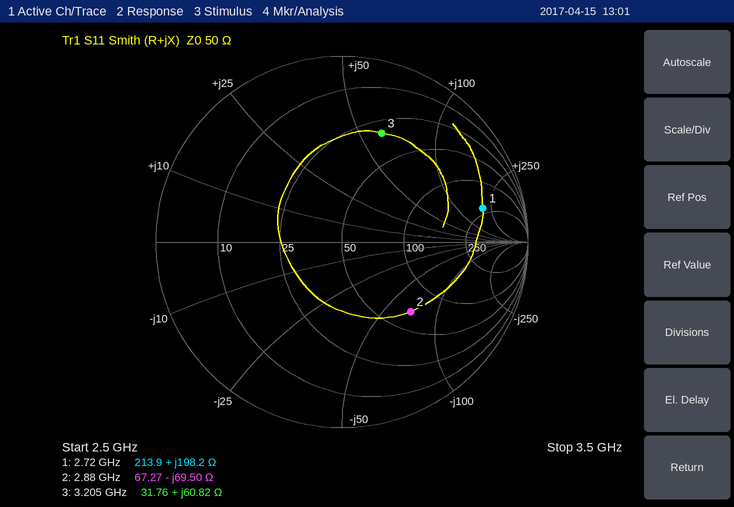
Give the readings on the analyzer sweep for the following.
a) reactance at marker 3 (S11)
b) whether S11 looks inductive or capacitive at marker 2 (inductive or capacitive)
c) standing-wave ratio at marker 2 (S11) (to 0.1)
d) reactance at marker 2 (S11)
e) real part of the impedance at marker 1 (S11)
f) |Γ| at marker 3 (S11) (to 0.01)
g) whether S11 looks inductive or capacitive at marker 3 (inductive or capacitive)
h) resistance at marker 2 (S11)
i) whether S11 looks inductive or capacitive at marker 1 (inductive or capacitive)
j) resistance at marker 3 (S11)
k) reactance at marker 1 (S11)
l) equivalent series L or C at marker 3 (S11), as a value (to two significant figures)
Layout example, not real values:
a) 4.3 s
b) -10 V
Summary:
a) +60.82 Ω
b) capacitive
c) 3.2
d) -69.50 Ω
e) 213.9 Ω
f) 0.62
g) inductive
h) 67.27 Ω
i) inductive
j) 31.76 Ω
k) +198.2 Ω
l) 3.0 nH
